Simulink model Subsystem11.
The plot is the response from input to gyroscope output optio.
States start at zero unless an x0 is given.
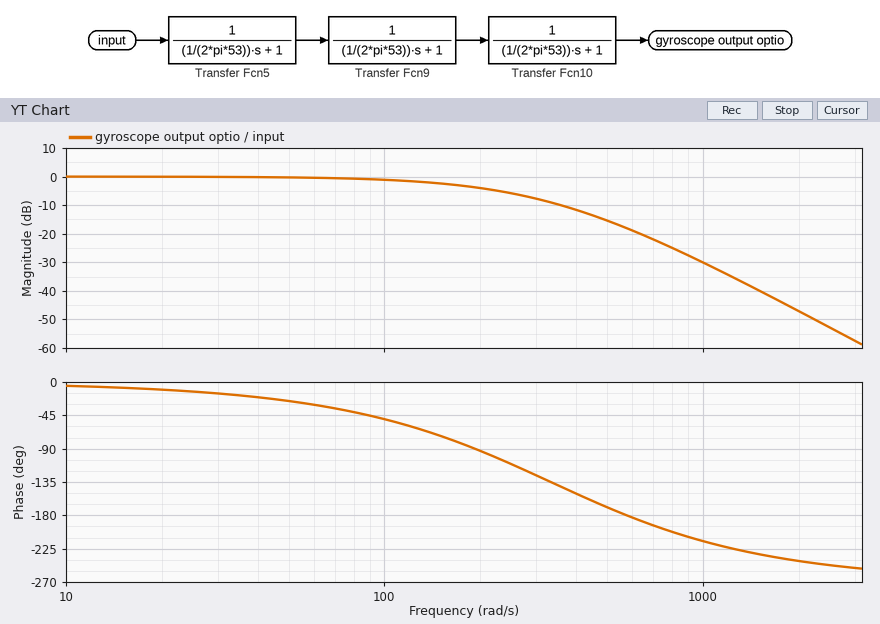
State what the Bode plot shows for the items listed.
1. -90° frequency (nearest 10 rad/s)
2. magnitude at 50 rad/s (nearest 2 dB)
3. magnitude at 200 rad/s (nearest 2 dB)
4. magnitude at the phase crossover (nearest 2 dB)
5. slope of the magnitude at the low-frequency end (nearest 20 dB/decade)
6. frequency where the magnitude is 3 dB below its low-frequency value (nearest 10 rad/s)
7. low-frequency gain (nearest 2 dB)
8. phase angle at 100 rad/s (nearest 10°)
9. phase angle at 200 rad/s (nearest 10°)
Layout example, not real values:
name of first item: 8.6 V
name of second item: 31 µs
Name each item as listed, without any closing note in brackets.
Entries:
-90° frequency: 190 rad/s
magnitude at 50 rad/s: 0 dB
magnitude at 200 rad/s: -4 dB
magnitude at the phase crossover: -18 dB
slope of the magnitude at the low-frequency end: 0 dB/decade
frequency where the magnitude is 3 dB below its low-frequency value: 170 rad/s
low-frequency gain: 0 dB
phase angle at 100 rad/s: -50°
phase angle at 200 rad/s: -90°
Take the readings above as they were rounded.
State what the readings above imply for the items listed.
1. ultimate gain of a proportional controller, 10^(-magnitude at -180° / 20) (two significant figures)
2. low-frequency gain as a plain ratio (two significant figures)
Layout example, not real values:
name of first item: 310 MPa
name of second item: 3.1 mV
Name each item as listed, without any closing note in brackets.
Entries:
ultimate gain of a proportional controller, 10^(-magnitude at -180° / 20): 7.9
low-frequency gain as a plain ratio: 1.0
